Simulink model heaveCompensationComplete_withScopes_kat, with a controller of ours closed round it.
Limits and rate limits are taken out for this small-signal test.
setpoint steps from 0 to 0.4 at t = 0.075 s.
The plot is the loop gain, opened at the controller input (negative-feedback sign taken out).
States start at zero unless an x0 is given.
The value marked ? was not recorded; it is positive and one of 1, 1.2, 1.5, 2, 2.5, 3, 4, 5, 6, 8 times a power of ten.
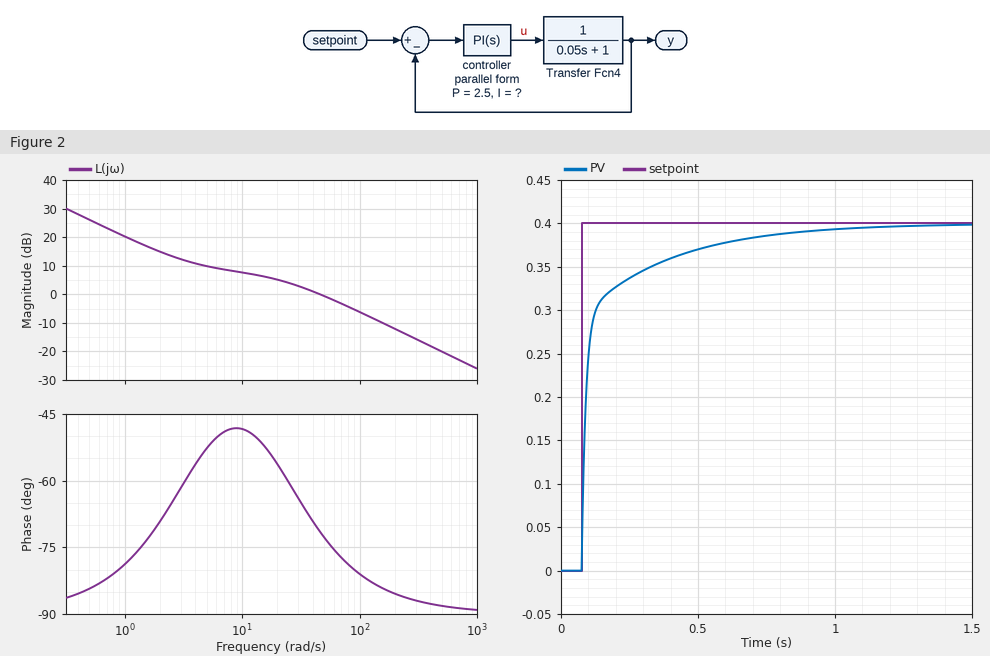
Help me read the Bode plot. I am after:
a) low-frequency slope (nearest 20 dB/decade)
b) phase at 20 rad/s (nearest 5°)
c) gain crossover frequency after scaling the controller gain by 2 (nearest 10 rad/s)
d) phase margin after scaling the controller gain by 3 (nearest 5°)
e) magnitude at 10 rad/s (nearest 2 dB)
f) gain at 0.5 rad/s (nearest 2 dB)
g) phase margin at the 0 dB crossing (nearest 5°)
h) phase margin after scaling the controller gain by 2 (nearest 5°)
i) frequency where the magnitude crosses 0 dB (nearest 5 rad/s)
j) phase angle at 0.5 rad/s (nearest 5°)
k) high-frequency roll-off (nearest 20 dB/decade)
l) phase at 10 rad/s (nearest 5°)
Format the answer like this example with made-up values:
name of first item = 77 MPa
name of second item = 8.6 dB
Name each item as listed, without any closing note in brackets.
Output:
low-frequency slope = -20 dB/decade
phase at 20 rad/s = -55°
gain crossover frequency after scaling the controller gain by 2 = 100 rad/s
phase margin after scaling the controller gain by 3 = 95°
magnitude at 10 rad/s = 8 dB
gain at 0.5 rad/s = 26 dB
phase margin at the 0 dB crossing = 110°
phase margin after scaling the controller gain by 2 = 100°
frequency where the magnitude crosses 0 dB = 45 rad/s
phase angle at 0.5 rad/s = -85°
high-frequency roll-off = -20 dB/decade
phase at 10 rad/s = -50°
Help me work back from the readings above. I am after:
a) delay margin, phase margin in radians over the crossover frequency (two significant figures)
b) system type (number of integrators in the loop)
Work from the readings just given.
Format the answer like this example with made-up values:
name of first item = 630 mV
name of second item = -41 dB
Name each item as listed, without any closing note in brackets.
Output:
delay margin, phase margin in radians over the crossover frequency = 0.043 s
system type = 1
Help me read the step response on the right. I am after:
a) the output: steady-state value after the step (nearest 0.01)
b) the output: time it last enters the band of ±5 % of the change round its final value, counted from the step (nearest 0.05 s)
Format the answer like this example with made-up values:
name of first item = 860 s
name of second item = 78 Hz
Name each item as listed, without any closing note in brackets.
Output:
the output: steady-state value after the step = 0.40
the output: time it last enters the band of ±5 % of the change round its final value, counted from the step = 0.55 s
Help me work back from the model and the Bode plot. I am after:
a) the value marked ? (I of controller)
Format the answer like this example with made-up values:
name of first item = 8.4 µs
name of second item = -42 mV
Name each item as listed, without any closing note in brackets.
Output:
the value marked ? = 10
